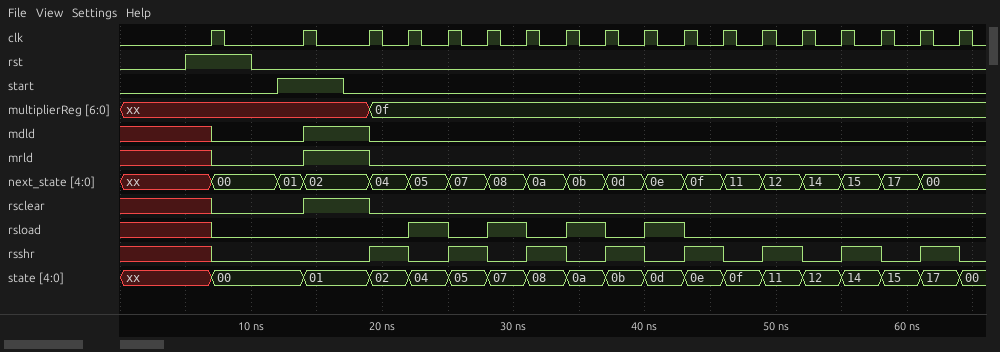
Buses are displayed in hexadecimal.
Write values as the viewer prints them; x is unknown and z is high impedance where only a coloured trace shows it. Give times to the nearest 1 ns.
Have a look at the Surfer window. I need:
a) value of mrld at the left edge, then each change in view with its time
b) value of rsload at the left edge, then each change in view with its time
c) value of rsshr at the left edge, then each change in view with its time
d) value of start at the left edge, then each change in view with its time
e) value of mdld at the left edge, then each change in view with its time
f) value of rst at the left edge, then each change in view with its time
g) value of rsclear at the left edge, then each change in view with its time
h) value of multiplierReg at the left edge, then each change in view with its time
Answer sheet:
x, 0 at 7 ns, 1 at 14 ns, 0 at 19 ns
x, 0 at 7 ns, 1 at 22 ns, 0 at 25 ns, 1 at 28 ns, 0 at 31 ns, 1 at 34 ns, 0 at 37 ns, 1 at 40 ns, 0 at 43 ns
x, 0 at 7 ns, 1 at 19 ns, 0 at 22 ns, 1 at 25 ns, 0 at 28 ns, 1 at 31 ns, 0 at 34 ns, 1 at 37 ns, 0 at 40 ns, 1 at 43 ns, 0 at 46 ns, 1 at 49 ns, 0 at 52 ns, 1 at 55 ns, 0 at 58 ns, 1 at 61 ns, 0 at 64 ns
0, 1 at 12 ns, 0 at 17 ns
x, 0 at 7 ns, 1 at 14 ns, 0 at 19 ns
0, 1 at 5 ns, 0 at 10 ns
x, 0 at 7 ns, 1 at 14 ns, 0 at 19 ns
xx, 0f at 19 ns
